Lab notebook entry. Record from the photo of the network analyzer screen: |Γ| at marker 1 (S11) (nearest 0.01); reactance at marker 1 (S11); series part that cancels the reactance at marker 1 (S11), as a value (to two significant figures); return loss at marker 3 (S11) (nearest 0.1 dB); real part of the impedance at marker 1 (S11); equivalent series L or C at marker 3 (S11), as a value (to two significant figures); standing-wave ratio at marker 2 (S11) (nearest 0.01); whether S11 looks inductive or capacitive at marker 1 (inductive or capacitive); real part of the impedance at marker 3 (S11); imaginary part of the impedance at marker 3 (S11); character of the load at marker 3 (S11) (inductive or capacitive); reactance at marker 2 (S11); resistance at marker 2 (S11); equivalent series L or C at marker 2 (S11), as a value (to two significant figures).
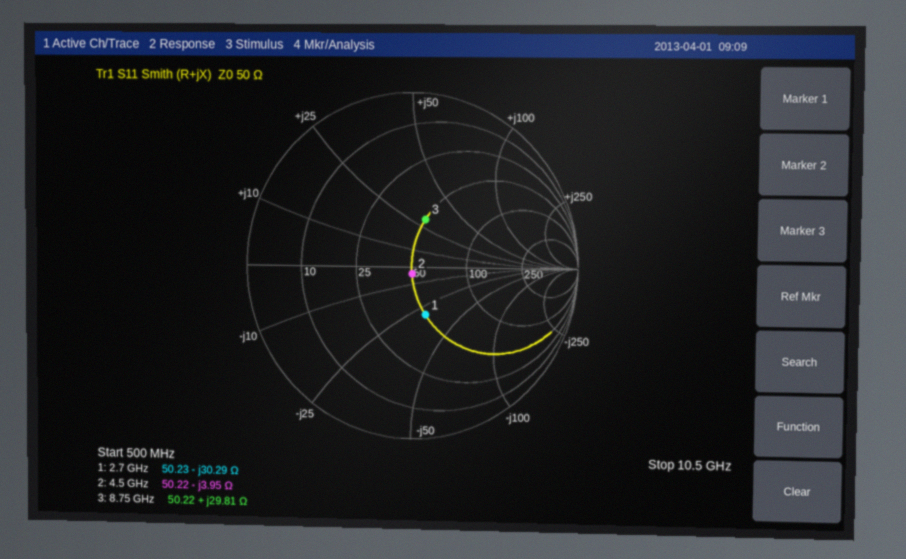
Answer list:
0.29
-30.29 Ω
1.8 nH
10.9 dB
50.23 Ω
540 pH
1.08
capacitive
50.22 Ω
+29.81 Ω
inductive
-3.95 Ω
50.22 Ω
9.0 pF
